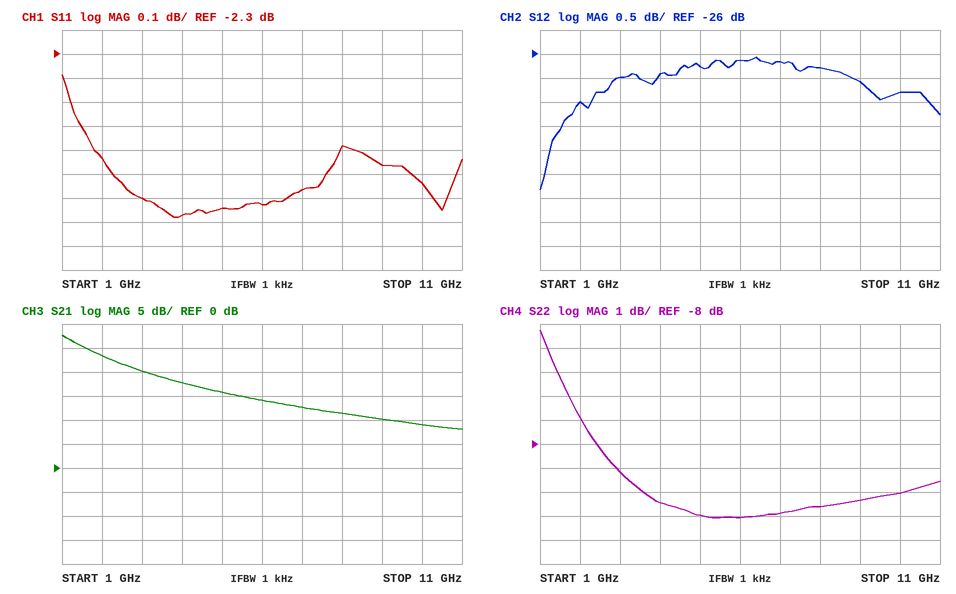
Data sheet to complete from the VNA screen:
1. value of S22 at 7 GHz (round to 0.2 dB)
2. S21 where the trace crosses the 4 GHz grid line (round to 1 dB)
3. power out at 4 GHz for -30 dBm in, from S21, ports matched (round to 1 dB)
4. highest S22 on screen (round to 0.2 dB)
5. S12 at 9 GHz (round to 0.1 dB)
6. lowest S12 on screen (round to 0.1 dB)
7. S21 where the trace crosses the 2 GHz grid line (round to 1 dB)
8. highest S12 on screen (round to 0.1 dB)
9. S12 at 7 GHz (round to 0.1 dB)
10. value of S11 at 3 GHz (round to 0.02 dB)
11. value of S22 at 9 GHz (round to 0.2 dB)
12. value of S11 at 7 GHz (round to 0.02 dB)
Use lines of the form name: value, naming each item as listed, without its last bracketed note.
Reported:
value of S22 at 7 GHz: -10.8 dB
S21 where the trace crosses the 4 GHz grid line: 18 dB
power out at 4 GHz for -30 dBm in, from S21, ports matched: -12 dBm
highest S22 on screen: -3.2 dB
S12 at 9 GHz: -26.6 dB
lowest S12 on screen: -28.8 dB
S21 where the trace crosses the 2 GHz grid line: 23 dB
highest S12 on screen: -26.1 dB
S12 at 7 GHz: -26.2 dB
value of S11 at 3 GHz: -2.90 dB
value of S22 at 9 GHz: -10.4 dB
value of S11 at 7 GHz: -2.86 dB
